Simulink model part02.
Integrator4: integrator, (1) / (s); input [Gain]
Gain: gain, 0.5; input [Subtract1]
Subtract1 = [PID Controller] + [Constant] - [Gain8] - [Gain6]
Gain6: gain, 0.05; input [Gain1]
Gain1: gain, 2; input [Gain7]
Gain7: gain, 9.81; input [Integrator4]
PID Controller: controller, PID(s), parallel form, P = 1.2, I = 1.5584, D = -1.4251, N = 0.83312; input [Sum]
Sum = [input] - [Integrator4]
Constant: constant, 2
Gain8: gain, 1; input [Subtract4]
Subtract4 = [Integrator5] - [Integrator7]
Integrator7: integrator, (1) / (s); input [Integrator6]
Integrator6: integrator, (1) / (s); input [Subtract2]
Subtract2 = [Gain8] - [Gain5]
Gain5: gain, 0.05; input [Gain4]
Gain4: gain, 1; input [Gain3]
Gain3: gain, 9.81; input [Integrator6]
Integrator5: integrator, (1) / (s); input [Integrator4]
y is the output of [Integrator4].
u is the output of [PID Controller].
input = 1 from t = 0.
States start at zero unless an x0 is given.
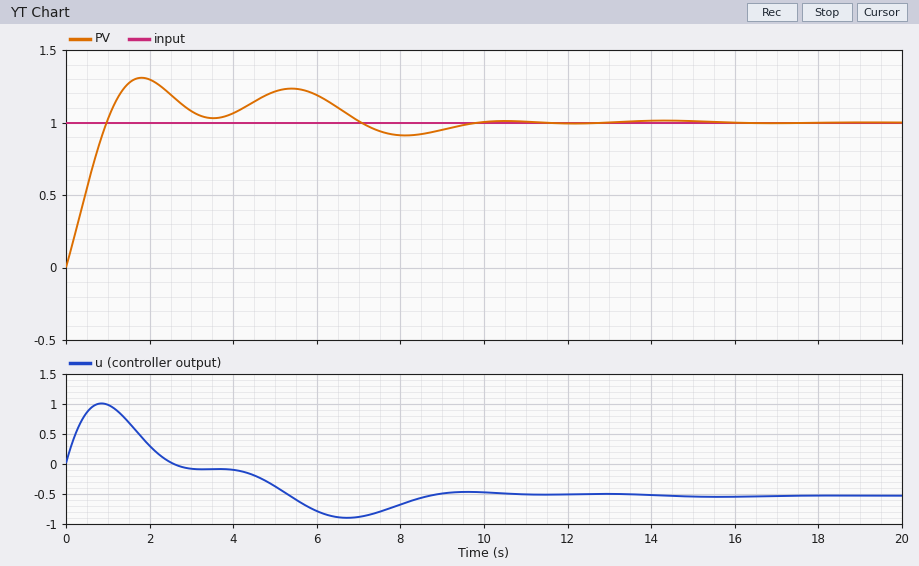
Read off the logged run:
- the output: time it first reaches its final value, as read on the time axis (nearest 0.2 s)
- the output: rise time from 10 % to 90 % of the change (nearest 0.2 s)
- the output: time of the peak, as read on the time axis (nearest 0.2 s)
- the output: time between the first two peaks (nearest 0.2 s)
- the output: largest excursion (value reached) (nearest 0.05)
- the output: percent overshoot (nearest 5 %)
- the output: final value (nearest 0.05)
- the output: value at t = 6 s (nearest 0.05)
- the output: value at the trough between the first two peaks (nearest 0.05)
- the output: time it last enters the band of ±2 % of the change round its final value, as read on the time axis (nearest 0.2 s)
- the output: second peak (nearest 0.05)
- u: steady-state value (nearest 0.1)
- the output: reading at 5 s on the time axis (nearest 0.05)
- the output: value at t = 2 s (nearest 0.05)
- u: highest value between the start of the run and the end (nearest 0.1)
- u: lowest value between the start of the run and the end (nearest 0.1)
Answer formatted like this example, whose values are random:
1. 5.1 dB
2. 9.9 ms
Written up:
1. 1.0 s
2. 0.8 s
3. 1.8 s
4. 3.6 s
5. 1.30
6. 30 %
7. 1.00
8. 1.20
9. 1.05
10. 9.4 s
11. 1.25
12. -0.5
13. 1.20
14. 1.30
15. 1.0
16. -0.9
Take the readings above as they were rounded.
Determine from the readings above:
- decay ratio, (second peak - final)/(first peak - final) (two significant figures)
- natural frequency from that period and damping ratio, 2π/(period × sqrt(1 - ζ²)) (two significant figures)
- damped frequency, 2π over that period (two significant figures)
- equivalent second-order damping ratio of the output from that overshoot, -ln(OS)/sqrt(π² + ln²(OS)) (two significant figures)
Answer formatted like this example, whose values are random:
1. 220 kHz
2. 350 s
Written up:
1. 0.83
2. 1.9 rad/s
3. 1.7 rad/s
4. 0.36
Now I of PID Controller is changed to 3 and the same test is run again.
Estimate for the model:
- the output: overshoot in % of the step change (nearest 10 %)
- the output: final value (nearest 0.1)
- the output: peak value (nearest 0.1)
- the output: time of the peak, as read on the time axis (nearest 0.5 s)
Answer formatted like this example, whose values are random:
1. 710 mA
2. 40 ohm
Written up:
1. 40 %
2. 1.0
3. 1.4
4. 1.5 s
